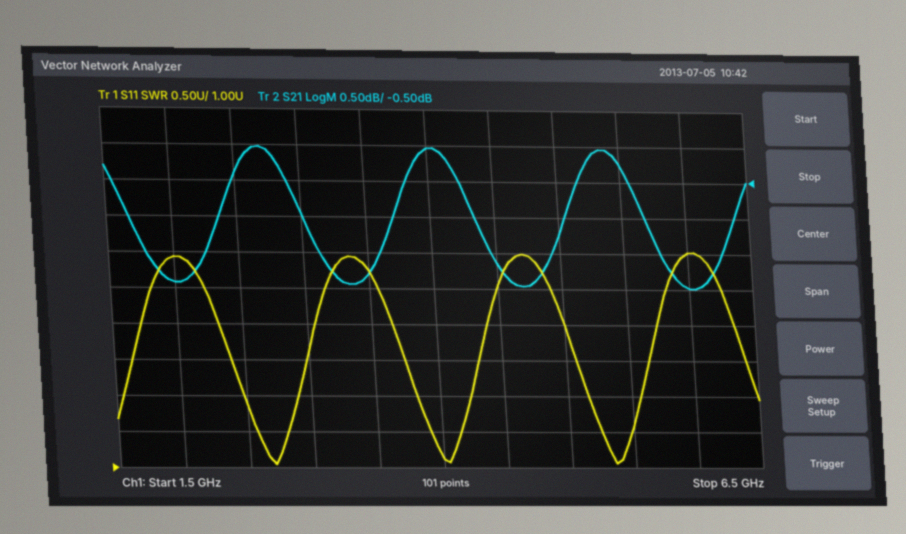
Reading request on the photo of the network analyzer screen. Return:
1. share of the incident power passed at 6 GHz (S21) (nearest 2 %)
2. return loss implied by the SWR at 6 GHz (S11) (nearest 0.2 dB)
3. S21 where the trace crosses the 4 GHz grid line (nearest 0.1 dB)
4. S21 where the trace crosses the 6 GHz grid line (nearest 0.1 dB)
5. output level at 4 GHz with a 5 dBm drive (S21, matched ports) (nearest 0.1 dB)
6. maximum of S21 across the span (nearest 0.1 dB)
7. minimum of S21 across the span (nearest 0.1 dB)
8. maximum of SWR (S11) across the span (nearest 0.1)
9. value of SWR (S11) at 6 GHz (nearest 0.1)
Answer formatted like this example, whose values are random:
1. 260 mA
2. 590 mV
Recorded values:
1. 64 %
2. 4.4 dB
3. 0.0 dB
4. -2.0 dB
5. 5.0 dBm
6. 0.0 dB
7. -2.0 dB
8. 4.0
9. 4.0
